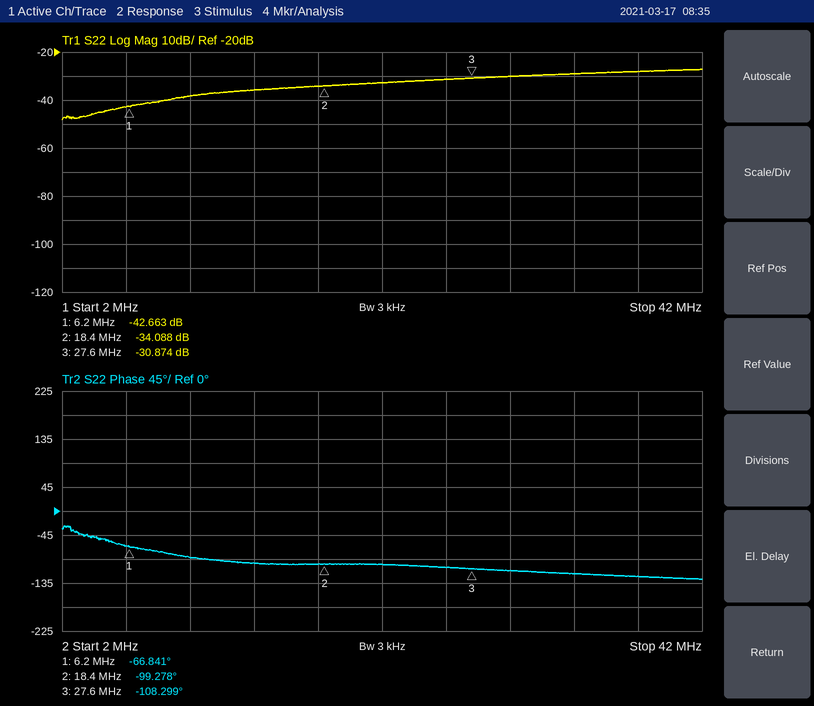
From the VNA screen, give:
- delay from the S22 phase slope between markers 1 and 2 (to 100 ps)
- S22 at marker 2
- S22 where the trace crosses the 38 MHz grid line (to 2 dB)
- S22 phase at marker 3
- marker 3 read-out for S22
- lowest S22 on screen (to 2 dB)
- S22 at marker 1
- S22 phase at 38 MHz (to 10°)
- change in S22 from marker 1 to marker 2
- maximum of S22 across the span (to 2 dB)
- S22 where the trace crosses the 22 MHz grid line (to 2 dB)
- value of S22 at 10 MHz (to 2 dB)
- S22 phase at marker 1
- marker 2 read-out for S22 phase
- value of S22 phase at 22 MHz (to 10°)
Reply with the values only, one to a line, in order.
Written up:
7.4 ns
-34.088 dB
-28 dB
-108.299°
-30.874 dB
-48 dB
-42.663 dB
-120°
8.575 dB
-28 dB
-32 dB
-38 dB
-66.841°
-99.278°
-100°
